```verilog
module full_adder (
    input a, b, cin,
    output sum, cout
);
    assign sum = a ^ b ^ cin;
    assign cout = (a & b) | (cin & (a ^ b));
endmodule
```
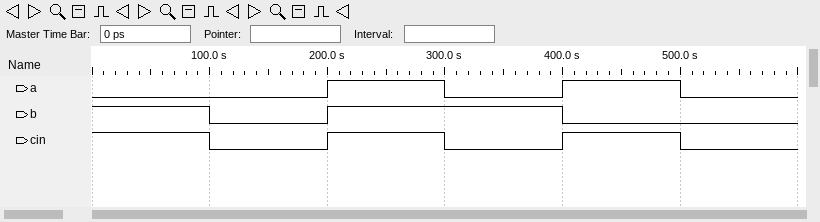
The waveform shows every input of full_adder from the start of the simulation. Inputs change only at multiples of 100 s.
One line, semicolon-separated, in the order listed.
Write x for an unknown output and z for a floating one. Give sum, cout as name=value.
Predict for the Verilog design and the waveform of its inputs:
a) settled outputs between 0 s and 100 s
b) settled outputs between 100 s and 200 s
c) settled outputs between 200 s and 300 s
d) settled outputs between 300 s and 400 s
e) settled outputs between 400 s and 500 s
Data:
sum=0, cout=1; sum=0, cout=0; sum=1, cout=1; sum=1, cout=0; sum=0, cout=1
